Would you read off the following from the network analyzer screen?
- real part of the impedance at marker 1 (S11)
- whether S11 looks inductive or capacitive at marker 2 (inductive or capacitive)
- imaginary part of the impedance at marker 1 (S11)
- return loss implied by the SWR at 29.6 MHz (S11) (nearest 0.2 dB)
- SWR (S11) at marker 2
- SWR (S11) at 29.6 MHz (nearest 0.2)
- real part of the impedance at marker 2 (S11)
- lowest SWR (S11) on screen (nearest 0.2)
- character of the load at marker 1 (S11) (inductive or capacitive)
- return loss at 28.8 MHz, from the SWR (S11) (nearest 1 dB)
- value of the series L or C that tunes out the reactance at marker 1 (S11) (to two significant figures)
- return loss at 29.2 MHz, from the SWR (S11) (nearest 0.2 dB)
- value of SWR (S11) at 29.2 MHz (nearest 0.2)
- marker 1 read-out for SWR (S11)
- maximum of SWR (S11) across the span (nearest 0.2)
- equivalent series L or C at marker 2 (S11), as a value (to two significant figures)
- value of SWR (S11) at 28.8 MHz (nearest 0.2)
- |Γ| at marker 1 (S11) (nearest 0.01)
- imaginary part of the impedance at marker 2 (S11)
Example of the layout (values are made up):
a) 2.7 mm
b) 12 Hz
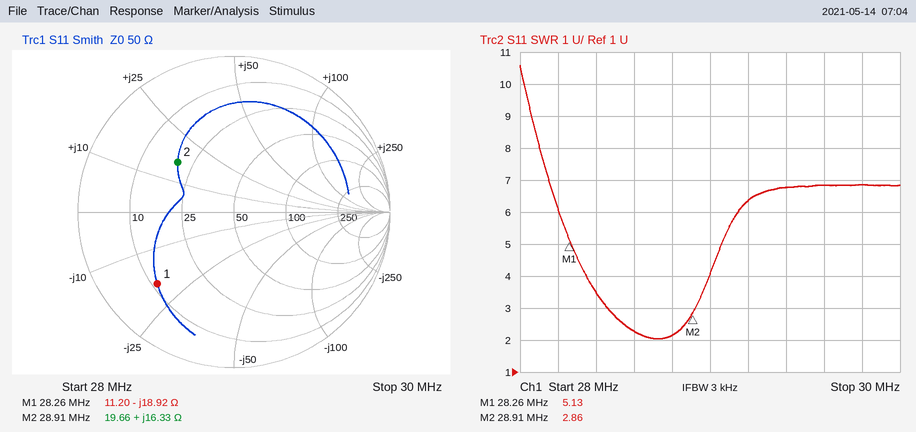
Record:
a) 11.20 Ω
b) inductive
c) -18.92 Ω
d) 2.6 dB
e) 2.86
f) 6.8
g) 19.66 Ω
h) 2.0
i) capacitive
j) 9 dB
k) 110 nH
l) 2.8 dB
m) 6.4
n) 5.13
o) 10.6
p) 90 nH
q) 2.2
r) 0.67
s) +16.33 Ω
